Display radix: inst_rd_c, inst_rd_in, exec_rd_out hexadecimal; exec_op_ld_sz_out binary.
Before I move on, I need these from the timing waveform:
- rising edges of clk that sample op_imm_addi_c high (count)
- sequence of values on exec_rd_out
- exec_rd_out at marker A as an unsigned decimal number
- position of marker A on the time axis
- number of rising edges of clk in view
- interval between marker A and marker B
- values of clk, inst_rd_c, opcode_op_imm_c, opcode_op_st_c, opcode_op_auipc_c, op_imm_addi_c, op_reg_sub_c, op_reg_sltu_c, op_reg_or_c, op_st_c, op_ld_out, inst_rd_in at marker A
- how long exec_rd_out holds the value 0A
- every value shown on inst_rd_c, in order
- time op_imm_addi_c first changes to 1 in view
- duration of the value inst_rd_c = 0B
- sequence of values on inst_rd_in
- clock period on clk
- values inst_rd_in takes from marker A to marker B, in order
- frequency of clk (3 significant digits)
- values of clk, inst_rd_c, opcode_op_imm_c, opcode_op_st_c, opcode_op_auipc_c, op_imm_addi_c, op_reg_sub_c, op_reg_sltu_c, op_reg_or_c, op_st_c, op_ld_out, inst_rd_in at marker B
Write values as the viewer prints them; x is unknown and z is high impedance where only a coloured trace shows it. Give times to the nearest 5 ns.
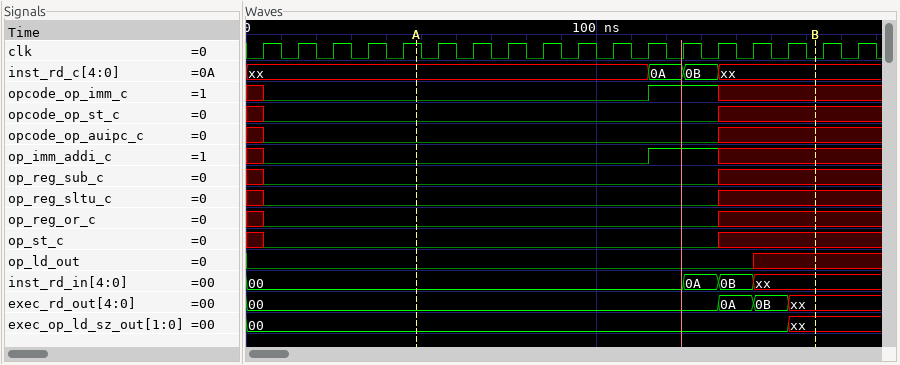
2
00, 0A, 0B, xx
0
50 ns
18
115 ns
clk=1, inst_rd_c=xx, opcode_op_imm_c=0, opcode_op_st_c=0, opcode_op_auipc_c=0, op_imm_addi_c=0, op_reg_sub_c=0, op_reg_sltu_c=0, op_reg_or_c=0, op_st_c=0, op_ld_out=0, inst_rd_in=00
10 ns
xx, 0A, 0B, xx
115 ns
10 ns
00, 0A, 0B, xx
10 ns
00, 0A, 0B, xx
100 MHz
clk=0, inst_rd_c=xx, opcode_op_imm_c=x, opcode_op_st_c=x, opcode_op_auipc_c=x, op_imm_addi_c=x, op_reg_sub_c=x, op_reg_sltu_c=x, op_reg_or_c=x, op_st_c=x, op_ld_out=x, inst_rd_in=xx
